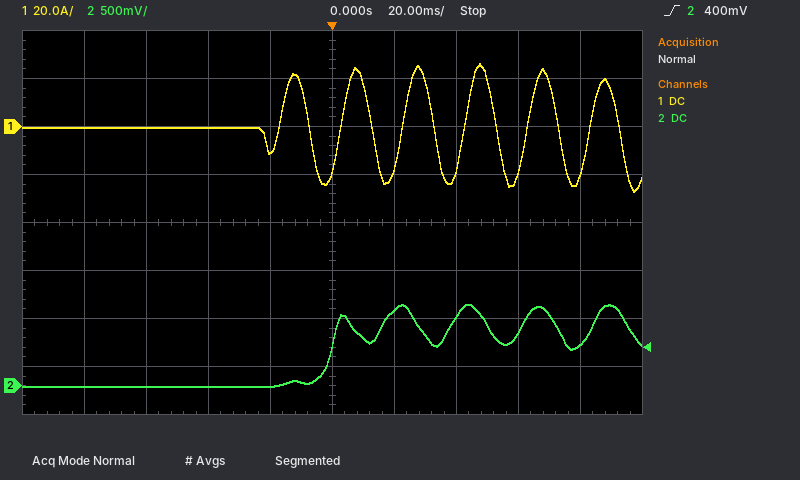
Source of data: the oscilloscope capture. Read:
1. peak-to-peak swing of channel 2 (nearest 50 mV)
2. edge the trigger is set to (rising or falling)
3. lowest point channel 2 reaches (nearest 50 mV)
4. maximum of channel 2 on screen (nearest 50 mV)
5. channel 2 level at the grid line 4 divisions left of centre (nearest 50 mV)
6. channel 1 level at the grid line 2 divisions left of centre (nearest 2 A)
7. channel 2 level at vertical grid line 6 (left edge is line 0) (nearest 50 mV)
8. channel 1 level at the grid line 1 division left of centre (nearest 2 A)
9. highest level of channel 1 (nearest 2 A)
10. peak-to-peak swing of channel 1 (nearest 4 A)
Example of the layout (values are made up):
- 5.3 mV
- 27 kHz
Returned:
- 850 mV
- rising
- 0 mV
- 850 mV
- 0 mV
- 0 A
- 800 mV
- -10 A
- 26 A
- 52 A
